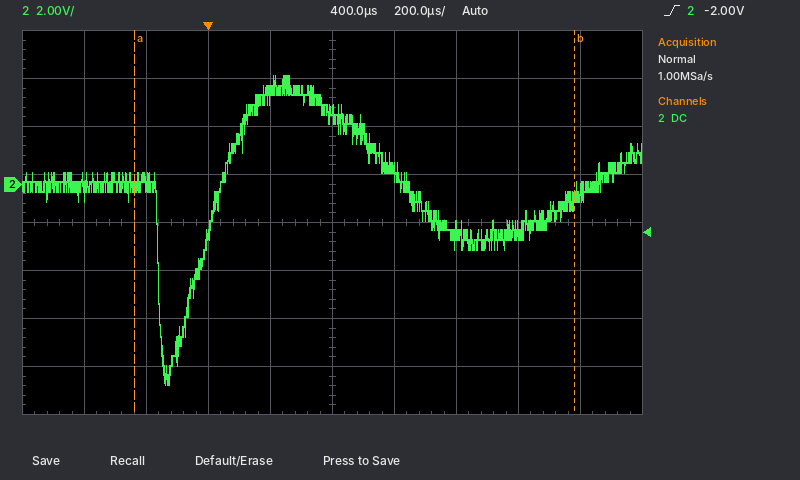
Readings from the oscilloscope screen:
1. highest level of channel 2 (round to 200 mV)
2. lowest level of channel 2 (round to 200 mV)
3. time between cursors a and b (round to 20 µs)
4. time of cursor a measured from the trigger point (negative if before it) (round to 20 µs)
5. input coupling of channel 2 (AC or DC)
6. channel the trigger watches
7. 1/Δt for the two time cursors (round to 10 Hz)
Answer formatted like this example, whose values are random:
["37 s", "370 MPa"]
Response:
["4.6 V", "-8.4 V", "1.42 ms", "-240 µs", "DC", "channel 2", "700 Hz"]
